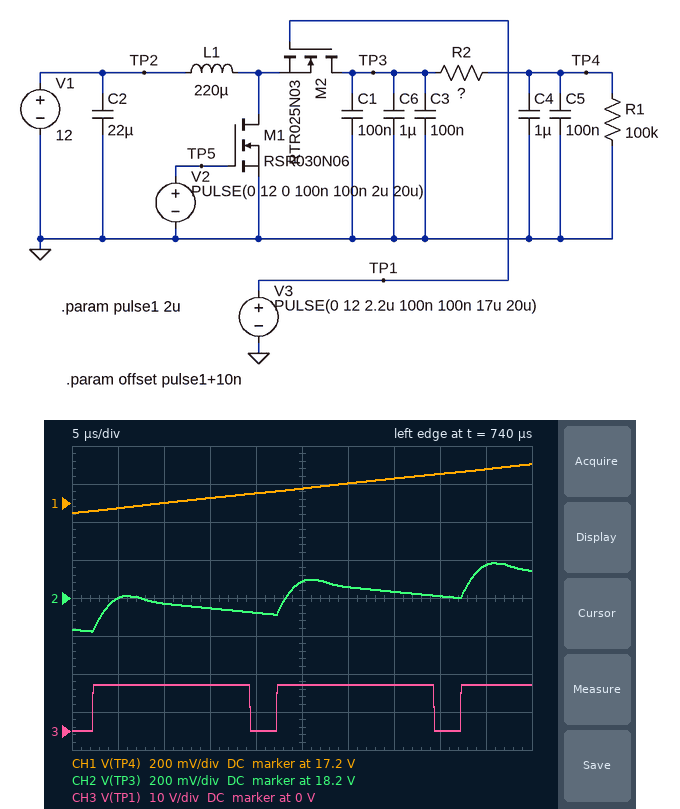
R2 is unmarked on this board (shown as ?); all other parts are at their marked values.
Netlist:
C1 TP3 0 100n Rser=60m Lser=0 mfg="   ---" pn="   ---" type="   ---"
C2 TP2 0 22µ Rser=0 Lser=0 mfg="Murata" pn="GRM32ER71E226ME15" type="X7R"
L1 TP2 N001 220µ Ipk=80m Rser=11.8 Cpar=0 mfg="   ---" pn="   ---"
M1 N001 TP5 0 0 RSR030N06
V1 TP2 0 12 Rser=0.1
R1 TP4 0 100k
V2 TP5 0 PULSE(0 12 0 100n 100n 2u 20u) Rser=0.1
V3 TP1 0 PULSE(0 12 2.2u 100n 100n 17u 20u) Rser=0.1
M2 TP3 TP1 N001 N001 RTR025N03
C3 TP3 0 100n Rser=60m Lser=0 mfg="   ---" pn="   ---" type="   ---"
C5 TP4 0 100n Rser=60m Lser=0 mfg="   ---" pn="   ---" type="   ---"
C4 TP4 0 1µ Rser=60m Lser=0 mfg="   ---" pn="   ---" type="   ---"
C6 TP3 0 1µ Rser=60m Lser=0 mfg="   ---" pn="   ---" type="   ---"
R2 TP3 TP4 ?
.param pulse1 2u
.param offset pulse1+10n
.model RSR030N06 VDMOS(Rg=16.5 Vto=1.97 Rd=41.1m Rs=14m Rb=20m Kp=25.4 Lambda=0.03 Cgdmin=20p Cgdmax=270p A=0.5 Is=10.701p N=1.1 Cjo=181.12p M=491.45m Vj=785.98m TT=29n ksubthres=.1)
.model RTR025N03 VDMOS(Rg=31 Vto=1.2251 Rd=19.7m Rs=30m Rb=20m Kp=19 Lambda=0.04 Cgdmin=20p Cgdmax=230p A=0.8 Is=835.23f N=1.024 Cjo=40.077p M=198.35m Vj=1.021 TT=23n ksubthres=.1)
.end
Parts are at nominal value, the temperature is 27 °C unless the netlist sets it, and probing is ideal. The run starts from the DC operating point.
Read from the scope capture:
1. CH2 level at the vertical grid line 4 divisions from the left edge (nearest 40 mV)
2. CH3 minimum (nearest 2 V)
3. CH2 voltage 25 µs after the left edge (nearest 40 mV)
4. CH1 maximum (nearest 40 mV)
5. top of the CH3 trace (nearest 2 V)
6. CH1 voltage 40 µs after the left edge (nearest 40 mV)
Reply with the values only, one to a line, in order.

18.12 V
0 V
18.28 V
17.40 V
12 V
17.36 V
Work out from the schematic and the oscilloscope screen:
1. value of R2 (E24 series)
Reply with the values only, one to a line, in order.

160 Ω
